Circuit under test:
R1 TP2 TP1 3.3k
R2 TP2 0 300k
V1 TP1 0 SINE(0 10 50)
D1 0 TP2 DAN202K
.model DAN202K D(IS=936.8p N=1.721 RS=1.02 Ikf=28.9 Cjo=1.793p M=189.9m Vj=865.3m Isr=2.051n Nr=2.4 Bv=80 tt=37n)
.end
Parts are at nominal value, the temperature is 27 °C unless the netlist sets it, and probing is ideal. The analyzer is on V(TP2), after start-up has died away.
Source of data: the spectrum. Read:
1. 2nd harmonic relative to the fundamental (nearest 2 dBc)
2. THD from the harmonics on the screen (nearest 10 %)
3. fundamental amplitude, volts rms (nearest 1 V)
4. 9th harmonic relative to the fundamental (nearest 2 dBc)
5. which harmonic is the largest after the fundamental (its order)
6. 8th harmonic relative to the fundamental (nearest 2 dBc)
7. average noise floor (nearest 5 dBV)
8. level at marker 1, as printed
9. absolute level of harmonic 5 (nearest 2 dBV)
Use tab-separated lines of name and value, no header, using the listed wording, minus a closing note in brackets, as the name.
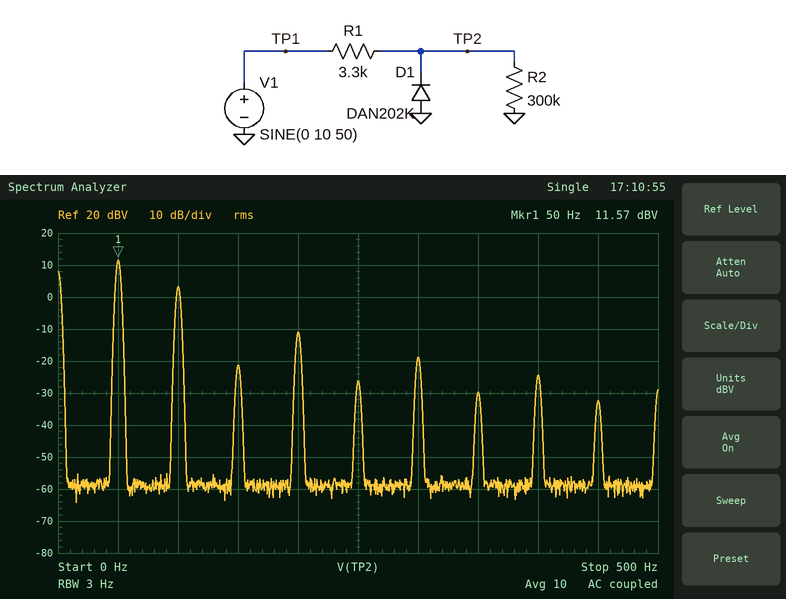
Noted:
2nd harmonic relative to the fundamental	-8 dBc
THD from the harmonics on the screen	40 %
fundamental amplitude, volts rms	4 V
9th harmonic relative to the fundamental	-44 dBc
which harmonic is the largest after the fundamental	2
8th harmonic relative to the fundamental	-36 dBc
average noise floor	-60 dBV
level at marker 1, as printed	11.57 dBV
absolute level of harmonic 5	-26 dBV
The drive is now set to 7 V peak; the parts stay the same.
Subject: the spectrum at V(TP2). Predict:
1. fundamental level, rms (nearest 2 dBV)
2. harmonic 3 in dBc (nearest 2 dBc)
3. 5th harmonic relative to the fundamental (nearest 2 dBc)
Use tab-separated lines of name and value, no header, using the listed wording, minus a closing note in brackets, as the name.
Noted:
fundamental level, rms	8 dBV
harmonic 3 in dBc	-30 dBc
5th harmonic relative to the fundamental	-36 dBc
